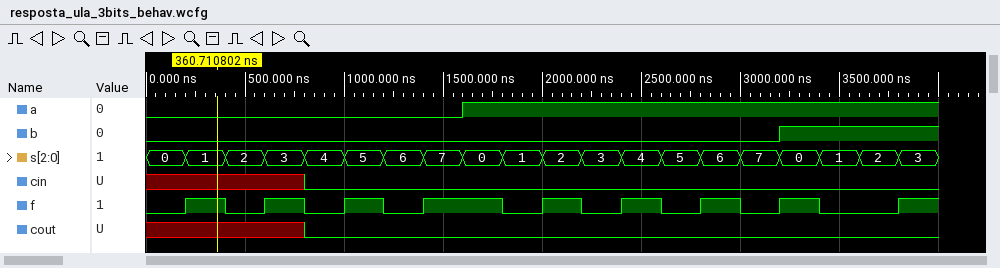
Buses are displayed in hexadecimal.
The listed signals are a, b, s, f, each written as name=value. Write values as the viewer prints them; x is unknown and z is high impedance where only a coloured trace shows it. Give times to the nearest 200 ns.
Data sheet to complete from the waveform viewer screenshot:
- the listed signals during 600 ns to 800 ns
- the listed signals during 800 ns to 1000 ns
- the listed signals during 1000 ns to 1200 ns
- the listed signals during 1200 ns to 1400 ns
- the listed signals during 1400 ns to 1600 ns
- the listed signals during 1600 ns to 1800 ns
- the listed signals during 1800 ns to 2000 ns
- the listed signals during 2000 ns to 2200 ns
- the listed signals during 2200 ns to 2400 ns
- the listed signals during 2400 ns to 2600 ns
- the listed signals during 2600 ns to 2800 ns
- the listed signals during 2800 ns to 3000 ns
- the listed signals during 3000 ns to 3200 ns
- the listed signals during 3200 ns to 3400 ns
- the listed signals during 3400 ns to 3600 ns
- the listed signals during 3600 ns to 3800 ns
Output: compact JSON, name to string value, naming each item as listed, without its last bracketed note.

{"the listed signals during 600 ns to 800 ns": "a=0, b=0, s=3, f=1", "the listed signals during 800 ns to 1000 ns": "a=0, b=0, s=4, f=0", "the listed signals during 1000 ns to 1200 ns": "a=0, b=0, s=5, f=1", "the listed signals during 1200 ns to 1400 ns": "a=0, b=0, s=6, f=0", "the listed signals during 1400 ns to 1600 ns": "a=0, b=0, s=7, f=1", "the listed signals during 1600 ns to 1800 ns": "a=1, b=0, s=0, f=1", "the listed signals during 1800 ns to 2000 ns": "a=1, b=0, s=1, f=0", "the listed signals during 2000 ns to 2200 ns": "a=1, b=0, s=2, f=1", "the listed signals during 2200 ns to 2400 ns": "a=1, b=0, s=3, f=0", "the listed signals during 2400 ns to 2600 ns": "a=1, b=0, s=4, f=1", "the listed signals during 2600 ns to 2800 ns": "a=1, b=0, s=5, f=0", "the listed signals during 2800 ns to 3000 ns": "a=1, b=0, s=6, f=1", "the listed signals during 3000 ns to 3200 ns": "a=1, b=0, s=7, f=0", "the listed signals during 3200 ns to 3400 ns": "a=1, b=1, s=0, f=1", "the listed signals during 3400 ns to 3600 ns": "a=1, b=1, s=1, f=0", "the listed signals during 3600 ns to 3800 ns": "a=1, b=1, s=2, f=0"}
